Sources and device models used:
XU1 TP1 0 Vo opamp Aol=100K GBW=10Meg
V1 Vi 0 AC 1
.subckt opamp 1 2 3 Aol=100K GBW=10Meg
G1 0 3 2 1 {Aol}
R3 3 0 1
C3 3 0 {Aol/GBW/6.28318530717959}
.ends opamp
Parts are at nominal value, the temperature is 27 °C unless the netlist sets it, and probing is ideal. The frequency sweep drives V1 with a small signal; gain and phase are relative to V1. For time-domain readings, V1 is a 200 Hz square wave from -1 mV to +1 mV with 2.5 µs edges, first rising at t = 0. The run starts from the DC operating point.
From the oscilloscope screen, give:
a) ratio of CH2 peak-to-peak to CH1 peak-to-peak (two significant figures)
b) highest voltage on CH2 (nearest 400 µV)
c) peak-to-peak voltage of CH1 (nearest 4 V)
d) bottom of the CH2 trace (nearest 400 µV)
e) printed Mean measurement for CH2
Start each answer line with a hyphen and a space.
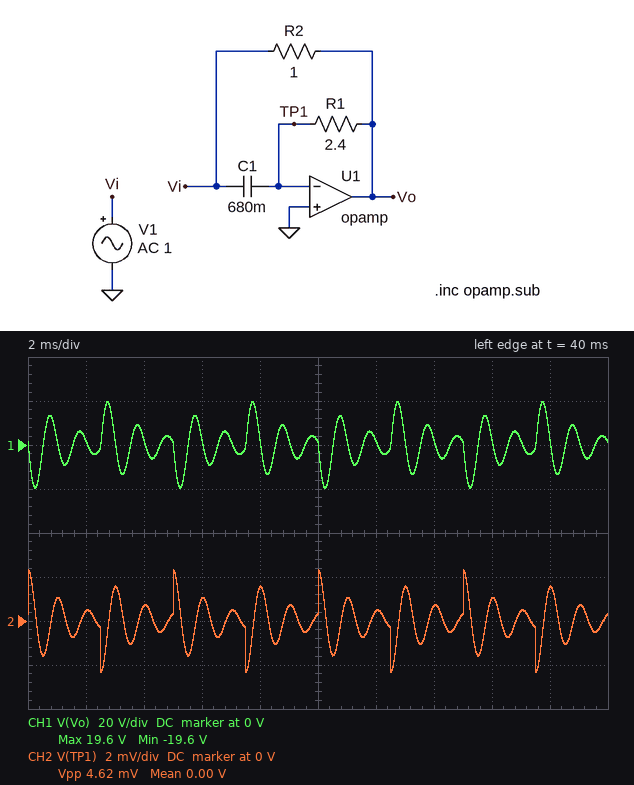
- 0.00012
- 2.4 mV
- 40 V
- -2.4 mV
- 0.00 V
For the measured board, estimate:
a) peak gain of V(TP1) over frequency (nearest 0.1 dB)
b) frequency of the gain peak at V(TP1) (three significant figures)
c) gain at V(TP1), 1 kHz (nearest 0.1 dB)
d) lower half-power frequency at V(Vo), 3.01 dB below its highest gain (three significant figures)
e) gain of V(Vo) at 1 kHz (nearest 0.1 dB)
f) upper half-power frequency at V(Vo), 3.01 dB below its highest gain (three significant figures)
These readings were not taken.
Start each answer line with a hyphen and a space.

- 12.5 dB
- 1.00 kHz
- 12.5 dB
- 874 Hz
- 92.3 dB
- 1.12 kHz
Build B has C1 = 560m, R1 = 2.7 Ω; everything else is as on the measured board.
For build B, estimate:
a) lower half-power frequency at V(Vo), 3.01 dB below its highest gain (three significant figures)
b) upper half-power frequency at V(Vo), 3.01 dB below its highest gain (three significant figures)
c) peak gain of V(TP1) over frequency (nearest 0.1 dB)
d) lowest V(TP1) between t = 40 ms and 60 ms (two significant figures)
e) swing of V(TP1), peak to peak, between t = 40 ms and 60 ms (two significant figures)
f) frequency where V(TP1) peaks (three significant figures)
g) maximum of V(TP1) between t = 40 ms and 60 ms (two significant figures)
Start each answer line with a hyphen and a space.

- 914 Hz
- 1.15 kHz
- 13.0 dB
- -2.4 mV
- 4.7 mV
- 1.04 kHz
- 2.4 mV
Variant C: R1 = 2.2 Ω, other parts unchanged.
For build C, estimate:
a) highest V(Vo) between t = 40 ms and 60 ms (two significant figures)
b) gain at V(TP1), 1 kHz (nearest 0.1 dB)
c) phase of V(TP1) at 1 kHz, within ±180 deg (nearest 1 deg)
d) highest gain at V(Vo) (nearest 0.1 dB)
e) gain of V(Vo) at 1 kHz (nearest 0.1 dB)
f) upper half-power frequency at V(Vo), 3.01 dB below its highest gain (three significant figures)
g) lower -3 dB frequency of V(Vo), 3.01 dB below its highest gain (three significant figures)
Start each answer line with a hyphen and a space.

- 19 V
- 12.2 dB
- 91 deg
- 92.2 dB
- 91.9 dB
- 1.16 kHz
- 916 Hz
